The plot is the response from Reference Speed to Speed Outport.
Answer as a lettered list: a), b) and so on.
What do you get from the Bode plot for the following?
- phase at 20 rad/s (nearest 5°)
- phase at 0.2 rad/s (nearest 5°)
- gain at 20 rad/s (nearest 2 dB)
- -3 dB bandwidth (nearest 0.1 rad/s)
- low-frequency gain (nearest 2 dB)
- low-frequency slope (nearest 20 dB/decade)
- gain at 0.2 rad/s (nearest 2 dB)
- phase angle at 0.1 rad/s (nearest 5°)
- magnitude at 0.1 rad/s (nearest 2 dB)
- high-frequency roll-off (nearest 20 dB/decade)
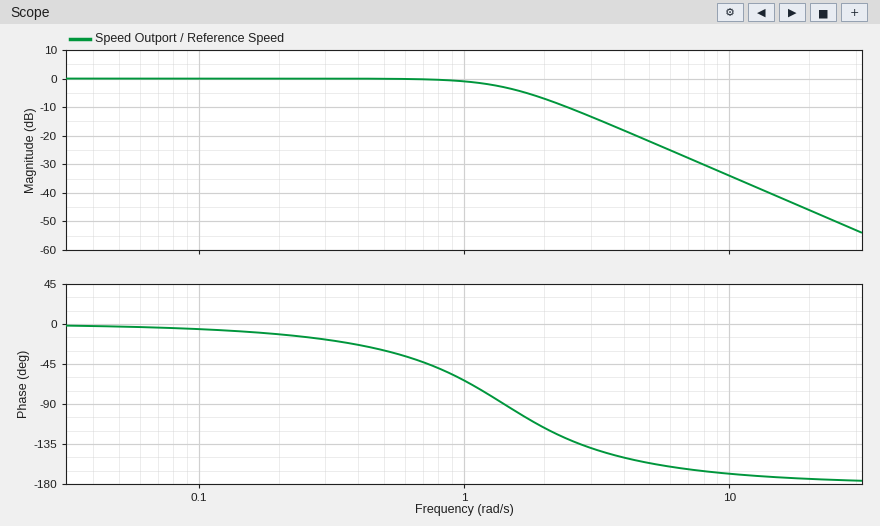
a) -175°
b) -10°
c) -46 dB
d) 1.4 rad/s
e) 0 dB
f) 0 dB/decade
g) 0 dB
h) -5°
i) 0 dB
j) -40 dB/decade
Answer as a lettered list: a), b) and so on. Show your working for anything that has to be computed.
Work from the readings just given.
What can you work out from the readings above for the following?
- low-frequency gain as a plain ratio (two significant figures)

a) 10^(0 / 20) = 1.0
